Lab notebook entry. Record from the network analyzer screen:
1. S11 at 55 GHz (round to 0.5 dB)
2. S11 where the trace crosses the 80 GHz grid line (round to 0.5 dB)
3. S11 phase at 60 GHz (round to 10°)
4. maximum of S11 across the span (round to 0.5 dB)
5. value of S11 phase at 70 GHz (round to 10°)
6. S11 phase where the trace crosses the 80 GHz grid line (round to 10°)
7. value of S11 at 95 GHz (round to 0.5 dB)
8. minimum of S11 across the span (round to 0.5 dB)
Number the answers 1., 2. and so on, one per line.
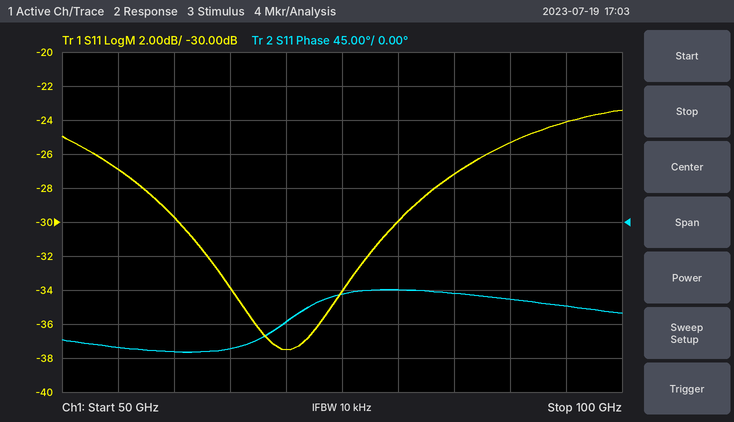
1. -27.0 dB
2. -30.0 dB
3. -170°
4. -23.5 dB
5. -130°
6. -90°
7. -24.0 dB
8. -37.5 dB
